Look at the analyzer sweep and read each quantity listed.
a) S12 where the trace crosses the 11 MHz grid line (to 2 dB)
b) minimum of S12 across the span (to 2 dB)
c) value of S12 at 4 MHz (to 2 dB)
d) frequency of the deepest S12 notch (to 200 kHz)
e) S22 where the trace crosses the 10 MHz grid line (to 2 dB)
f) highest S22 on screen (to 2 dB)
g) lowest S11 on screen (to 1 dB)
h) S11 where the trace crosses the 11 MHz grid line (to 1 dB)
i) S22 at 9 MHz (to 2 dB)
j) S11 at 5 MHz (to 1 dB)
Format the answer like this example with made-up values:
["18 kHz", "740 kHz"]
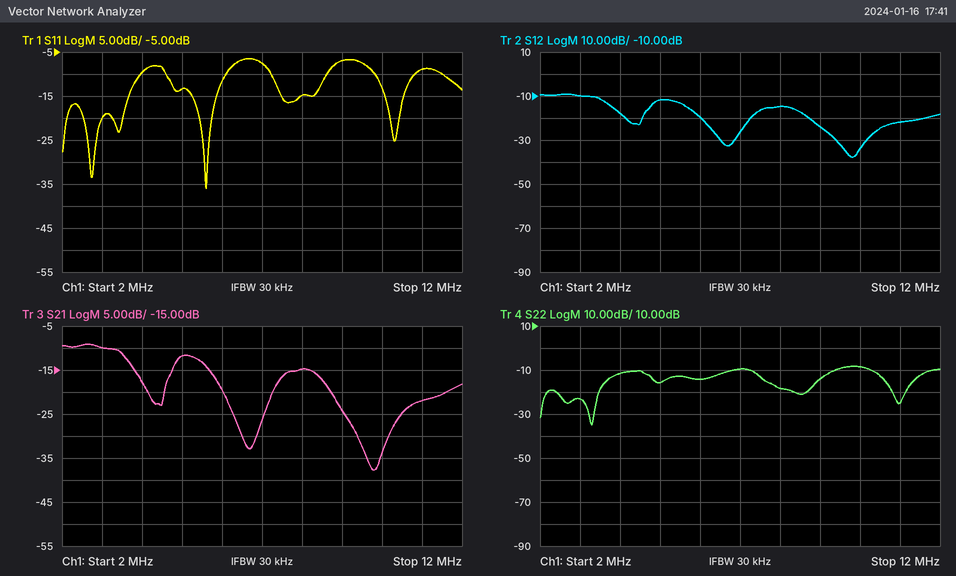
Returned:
["-22 dB", "-38 dB", "-18 dB", "9.8 MHz", "-8 dB", "-8 dB", "-36 dB", "-9 dB", "-14 dB", "-13 dB"]
